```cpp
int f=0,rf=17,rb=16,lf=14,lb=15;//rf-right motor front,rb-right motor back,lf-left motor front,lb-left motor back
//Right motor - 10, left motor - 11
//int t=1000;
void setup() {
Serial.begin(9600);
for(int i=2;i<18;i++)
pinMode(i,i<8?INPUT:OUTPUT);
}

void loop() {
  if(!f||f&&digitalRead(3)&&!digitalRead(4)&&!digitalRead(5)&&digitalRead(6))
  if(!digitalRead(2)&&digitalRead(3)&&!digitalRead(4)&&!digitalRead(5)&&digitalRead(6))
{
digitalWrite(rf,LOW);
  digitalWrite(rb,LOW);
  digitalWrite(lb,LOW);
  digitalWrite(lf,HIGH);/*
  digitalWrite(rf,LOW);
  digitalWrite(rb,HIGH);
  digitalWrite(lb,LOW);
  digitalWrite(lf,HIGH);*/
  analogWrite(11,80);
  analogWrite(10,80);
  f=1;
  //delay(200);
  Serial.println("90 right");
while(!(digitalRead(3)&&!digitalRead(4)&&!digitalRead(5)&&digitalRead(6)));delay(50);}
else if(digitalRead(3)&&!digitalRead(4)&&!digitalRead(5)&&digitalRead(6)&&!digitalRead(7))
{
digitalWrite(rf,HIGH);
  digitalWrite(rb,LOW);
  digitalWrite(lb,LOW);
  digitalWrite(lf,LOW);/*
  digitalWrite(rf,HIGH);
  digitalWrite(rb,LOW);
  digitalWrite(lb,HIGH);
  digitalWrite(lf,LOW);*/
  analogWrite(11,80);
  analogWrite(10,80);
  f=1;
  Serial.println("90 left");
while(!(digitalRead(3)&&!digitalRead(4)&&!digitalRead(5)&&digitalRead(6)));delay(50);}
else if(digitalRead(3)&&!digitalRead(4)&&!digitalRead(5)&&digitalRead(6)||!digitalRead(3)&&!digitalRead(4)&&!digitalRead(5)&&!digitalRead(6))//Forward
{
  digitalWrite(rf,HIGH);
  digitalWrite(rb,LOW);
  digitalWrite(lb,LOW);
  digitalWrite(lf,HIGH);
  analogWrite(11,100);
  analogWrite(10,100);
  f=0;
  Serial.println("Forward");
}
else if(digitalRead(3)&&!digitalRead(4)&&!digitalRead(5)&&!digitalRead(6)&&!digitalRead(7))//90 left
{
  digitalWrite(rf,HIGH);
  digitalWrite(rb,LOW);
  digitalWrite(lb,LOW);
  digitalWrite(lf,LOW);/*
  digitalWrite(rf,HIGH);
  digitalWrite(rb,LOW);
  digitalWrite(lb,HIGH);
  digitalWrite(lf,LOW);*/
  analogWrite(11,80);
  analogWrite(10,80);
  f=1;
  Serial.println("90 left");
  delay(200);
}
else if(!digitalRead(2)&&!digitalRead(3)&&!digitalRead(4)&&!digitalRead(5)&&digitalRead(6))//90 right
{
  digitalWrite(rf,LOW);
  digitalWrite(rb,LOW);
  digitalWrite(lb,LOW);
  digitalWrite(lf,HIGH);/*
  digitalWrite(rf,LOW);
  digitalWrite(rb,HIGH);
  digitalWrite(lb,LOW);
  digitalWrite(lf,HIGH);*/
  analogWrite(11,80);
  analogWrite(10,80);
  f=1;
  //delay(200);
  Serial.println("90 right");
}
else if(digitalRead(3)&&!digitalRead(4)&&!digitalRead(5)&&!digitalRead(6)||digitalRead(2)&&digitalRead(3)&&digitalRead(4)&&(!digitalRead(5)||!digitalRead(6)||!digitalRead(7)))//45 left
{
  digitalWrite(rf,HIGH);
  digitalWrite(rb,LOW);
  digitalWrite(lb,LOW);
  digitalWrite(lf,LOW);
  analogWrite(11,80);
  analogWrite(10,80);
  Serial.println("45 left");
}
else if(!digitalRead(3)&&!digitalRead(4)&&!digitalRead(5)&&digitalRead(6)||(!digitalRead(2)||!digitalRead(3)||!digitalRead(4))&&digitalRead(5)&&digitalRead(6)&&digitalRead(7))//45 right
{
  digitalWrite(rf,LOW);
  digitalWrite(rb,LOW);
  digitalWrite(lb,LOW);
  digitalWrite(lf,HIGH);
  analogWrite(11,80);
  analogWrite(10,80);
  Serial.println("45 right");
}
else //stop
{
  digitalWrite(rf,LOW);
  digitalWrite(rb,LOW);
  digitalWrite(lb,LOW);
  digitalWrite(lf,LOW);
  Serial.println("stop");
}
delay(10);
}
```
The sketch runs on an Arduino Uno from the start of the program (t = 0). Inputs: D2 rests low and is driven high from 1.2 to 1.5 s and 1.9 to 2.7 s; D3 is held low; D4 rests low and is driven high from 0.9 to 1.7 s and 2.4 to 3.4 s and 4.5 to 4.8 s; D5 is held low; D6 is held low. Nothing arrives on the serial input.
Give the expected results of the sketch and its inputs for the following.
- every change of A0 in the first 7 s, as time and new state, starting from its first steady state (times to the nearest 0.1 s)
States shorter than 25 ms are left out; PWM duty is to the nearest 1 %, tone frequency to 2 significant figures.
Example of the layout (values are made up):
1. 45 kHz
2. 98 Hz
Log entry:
1. 0 s high; 0.9 s low; 1.7 s high; 2.4 s low; 3.4 s high; 4.5 s low; 4.8 s high
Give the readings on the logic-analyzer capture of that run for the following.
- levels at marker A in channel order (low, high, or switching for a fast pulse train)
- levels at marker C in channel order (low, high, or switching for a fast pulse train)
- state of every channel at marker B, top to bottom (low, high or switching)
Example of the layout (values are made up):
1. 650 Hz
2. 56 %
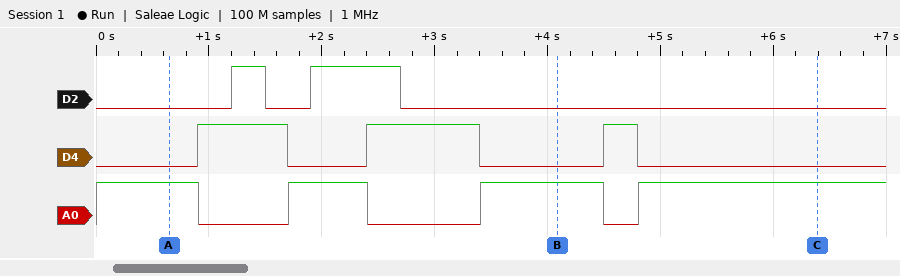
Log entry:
1. D2 low, D4 low, A0 high
2. D2 low, D4 low, A0 high
3. D2 low, D4 low, A0 high
